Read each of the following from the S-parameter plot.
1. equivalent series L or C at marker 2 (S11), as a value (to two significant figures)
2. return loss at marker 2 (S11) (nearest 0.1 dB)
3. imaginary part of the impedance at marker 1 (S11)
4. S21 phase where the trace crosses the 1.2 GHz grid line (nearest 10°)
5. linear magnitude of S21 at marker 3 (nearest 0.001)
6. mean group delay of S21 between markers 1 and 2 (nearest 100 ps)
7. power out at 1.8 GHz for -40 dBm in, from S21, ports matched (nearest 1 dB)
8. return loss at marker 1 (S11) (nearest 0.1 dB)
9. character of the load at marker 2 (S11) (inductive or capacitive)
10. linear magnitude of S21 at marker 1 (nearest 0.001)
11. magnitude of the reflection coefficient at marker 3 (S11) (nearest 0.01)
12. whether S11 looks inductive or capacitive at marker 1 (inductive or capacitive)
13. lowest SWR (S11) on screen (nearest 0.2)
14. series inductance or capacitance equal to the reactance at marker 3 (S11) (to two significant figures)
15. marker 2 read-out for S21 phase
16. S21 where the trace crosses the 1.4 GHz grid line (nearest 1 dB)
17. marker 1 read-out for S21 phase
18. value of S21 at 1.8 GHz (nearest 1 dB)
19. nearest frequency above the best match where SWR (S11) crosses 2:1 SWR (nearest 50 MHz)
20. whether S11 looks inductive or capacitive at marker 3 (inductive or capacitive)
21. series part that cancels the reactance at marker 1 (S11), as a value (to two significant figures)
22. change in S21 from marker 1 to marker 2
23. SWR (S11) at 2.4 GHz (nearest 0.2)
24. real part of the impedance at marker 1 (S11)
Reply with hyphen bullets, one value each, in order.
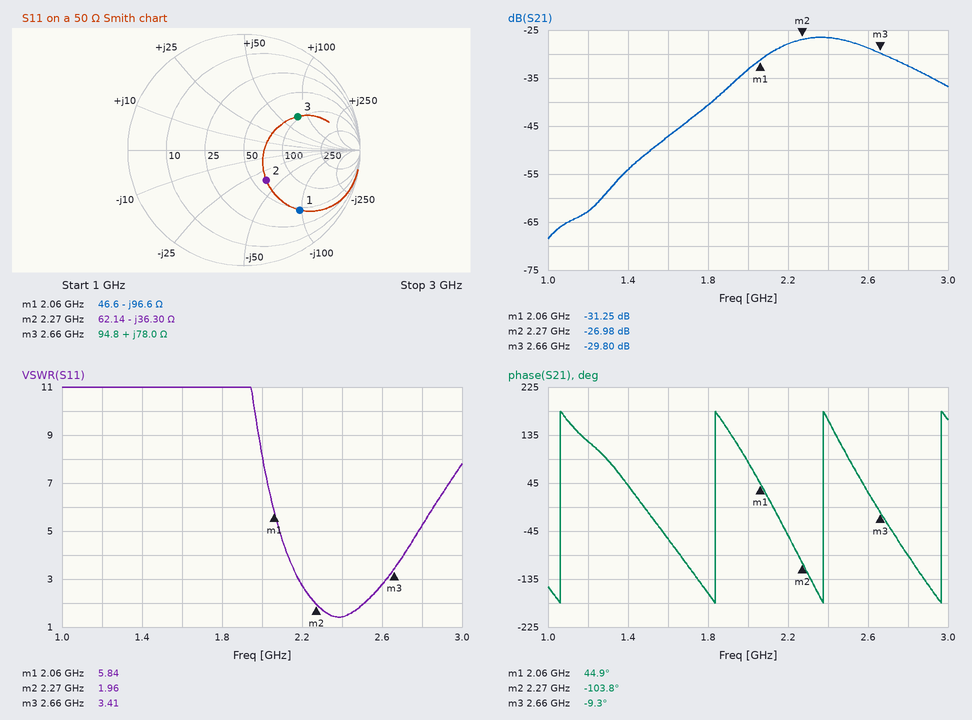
- 1.9 pF
- 9.8 dB
- -96.6 Ω
- 120°
- 0.032
- 2.0 ns
- -81 dBm
- 3.0 dB
- capacitive
- 0.027
- 0.55
- capacitive
- 1.4
- 4.7 nH
- -103.8°
- -54 dB
- 44.9°
- -41 dB
- 2.50 GHz
- inductive
- 7.5 nH
- 4.27 dB
- 1.4
- 46.6 Ω
